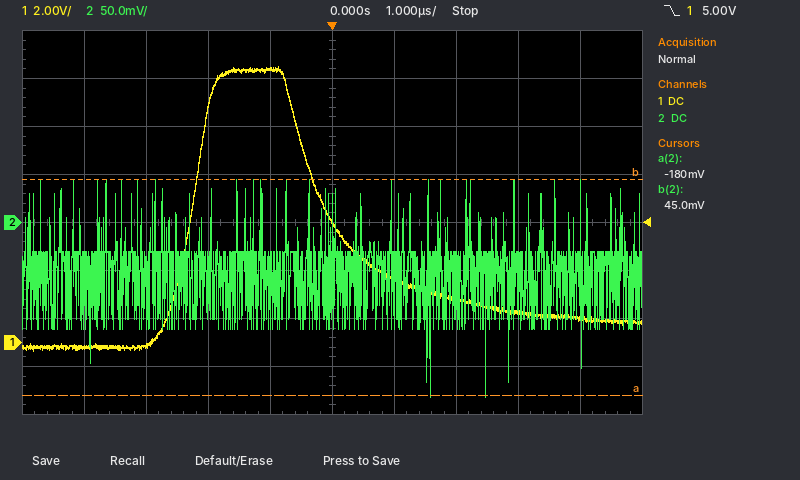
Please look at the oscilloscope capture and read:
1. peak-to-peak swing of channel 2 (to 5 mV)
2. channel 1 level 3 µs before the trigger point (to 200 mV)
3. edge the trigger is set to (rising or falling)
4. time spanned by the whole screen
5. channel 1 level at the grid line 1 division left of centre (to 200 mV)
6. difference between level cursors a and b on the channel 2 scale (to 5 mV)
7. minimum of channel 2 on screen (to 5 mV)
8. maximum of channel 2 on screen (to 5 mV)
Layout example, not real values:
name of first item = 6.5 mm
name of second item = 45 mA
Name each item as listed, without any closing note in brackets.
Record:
peak-to-peak swing of channel 2 = 225 mV
channel 1 level 3 µs before the trigger point = -200 mV
edge the trigger is set to = falling
time spanned by the whole screen = 10 µs
channel 1 level at the grid line 1 division left of centre = 11.4 V
difference between level cursors a and b on the channel 2 scale = 225 mV
minimum of channel 2 on screen = -180 mV
maximum of channel 2 on screen = 45 mV
